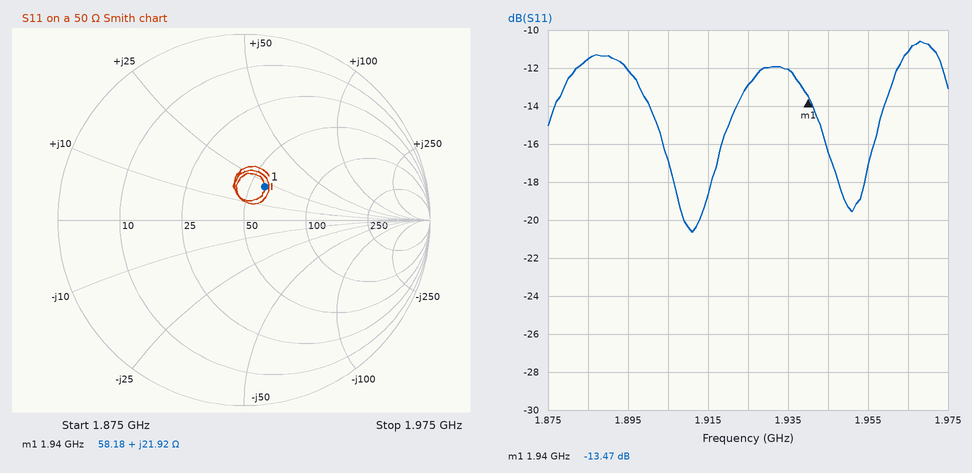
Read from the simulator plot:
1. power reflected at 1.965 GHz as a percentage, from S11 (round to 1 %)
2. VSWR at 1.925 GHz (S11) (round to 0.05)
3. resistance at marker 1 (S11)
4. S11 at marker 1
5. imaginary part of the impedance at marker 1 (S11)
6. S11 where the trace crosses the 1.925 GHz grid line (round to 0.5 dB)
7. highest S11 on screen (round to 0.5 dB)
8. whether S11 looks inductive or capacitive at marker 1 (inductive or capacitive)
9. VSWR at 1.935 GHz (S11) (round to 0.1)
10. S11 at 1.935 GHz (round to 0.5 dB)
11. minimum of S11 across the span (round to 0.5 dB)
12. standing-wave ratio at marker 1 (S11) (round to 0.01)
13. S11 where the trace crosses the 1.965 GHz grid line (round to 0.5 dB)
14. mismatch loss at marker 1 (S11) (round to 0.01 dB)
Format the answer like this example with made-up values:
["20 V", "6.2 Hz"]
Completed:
["8 %", "1.60", "58.18 Ω", "-13.47 dB", "+21.92 Ω", "-13.0 dB", "-10.5 dB", "inductive", "1.7", "-12.0 dB", "-20.5 dB", "1.54", "-11.0 dB", "0.20 dB"]
